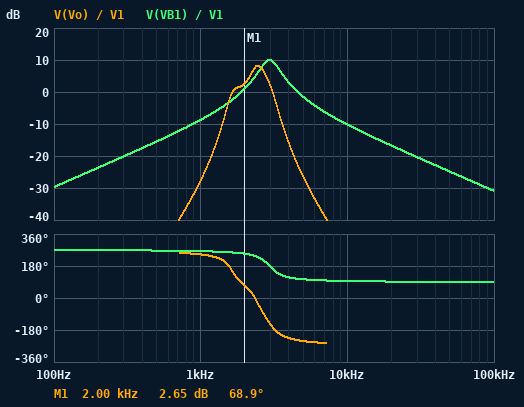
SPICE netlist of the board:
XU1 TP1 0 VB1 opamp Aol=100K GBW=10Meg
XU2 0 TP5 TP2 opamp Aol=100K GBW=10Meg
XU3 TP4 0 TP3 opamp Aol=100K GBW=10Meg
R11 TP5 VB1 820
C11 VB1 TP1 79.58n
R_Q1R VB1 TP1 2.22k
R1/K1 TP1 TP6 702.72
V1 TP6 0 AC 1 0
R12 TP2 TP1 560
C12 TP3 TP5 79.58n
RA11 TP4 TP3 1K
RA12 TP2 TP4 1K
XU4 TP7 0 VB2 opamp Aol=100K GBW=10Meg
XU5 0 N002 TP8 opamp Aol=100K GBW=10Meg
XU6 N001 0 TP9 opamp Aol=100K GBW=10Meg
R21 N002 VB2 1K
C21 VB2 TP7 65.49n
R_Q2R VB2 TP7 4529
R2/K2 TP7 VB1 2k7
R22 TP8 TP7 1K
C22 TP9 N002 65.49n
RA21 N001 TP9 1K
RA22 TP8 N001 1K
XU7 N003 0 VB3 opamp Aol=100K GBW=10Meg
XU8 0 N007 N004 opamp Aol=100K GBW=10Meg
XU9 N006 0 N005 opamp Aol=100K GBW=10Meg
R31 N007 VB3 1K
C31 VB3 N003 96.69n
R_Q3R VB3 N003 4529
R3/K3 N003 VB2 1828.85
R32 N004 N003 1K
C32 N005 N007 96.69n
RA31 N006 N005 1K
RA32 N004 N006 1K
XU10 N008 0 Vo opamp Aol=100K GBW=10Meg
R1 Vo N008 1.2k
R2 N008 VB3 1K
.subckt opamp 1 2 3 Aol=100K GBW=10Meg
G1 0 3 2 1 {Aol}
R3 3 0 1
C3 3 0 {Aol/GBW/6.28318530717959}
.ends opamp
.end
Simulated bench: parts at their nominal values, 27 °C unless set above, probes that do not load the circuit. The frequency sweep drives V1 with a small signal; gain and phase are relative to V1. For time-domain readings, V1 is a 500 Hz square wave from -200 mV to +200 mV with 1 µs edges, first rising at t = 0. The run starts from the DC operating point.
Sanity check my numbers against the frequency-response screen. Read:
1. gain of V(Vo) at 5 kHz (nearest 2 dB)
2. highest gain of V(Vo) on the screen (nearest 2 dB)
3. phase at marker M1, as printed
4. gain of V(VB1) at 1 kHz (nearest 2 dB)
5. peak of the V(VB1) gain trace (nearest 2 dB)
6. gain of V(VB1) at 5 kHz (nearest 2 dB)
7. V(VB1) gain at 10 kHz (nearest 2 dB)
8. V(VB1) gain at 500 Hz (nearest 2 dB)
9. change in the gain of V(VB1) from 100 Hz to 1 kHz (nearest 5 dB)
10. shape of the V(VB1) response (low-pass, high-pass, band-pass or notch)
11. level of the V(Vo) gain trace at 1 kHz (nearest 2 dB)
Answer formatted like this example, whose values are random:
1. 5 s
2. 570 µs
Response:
1. -26 dB
2. 8 dB
3. 68.9 deg
4. -8 dB
5. 10 dB
6. -2 dB
7. -10 dB
8. -16 dB
9. 20 dB
10. band-pass
11. -28 dB
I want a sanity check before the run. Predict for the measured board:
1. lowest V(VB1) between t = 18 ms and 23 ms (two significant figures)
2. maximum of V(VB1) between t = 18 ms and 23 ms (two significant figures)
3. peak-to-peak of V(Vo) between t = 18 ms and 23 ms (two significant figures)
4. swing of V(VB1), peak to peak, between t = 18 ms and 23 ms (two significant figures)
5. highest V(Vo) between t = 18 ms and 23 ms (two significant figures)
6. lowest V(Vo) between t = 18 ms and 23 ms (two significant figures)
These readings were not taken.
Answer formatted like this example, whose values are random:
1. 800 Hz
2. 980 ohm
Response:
1. -300 mV
2. 300 mV
3. 350 mV
4. 590 mV
5. 180 mV
6. -180 mV
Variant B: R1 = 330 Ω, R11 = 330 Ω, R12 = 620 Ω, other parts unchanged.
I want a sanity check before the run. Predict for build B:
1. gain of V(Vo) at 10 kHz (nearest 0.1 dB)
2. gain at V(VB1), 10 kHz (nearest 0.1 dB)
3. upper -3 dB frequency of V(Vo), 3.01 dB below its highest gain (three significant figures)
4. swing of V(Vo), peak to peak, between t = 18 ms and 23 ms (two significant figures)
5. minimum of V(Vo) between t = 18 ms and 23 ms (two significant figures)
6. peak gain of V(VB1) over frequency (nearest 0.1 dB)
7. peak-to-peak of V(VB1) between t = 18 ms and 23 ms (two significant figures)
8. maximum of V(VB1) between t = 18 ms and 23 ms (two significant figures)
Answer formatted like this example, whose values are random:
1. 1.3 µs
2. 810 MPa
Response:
1. -59.8 dB
2. -9.1 dB
3. 2.69 kHz
4. 25 mV
5. -13 mV
6. 10.0 dB
7. 460 mV
8. 230 mV
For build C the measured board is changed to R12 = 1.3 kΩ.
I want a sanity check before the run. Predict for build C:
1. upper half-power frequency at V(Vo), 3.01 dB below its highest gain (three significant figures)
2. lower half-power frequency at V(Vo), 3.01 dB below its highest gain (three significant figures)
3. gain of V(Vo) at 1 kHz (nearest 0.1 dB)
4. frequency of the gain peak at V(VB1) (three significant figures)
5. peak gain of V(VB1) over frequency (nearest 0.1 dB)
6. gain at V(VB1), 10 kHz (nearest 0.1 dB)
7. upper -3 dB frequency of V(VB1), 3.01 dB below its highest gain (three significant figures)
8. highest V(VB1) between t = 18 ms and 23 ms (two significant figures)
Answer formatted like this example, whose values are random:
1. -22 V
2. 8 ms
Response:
1. 2.46 kHz
2. 1.59 kHz
3. -19.1 dB
4. 1.94 kHz
5. 10.0 dB
6. -10.6 dB
7. 2.44 kHz
8. 410 mV
